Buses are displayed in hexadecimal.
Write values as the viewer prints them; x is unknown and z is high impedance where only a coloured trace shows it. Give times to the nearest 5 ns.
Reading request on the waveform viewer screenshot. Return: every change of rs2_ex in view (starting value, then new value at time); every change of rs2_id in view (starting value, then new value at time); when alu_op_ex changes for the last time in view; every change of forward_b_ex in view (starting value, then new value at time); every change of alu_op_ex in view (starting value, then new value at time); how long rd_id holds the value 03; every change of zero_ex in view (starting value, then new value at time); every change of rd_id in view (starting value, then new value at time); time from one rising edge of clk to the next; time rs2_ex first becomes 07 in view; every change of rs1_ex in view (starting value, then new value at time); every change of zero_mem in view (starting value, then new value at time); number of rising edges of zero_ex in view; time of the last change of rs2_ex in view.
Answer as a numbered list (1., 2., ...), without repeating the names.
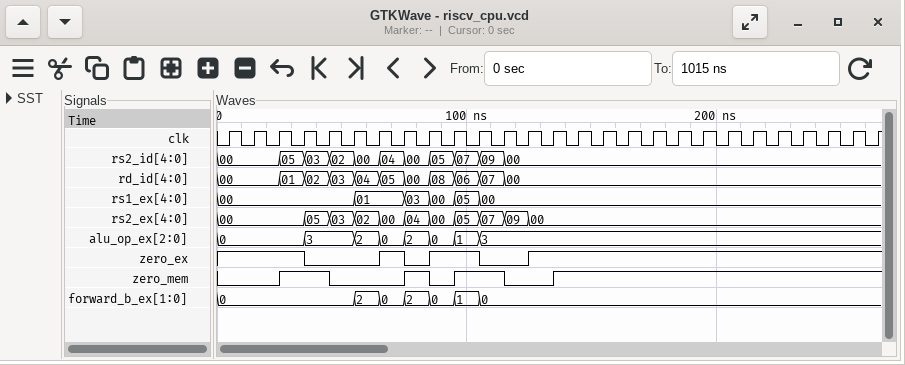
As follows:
1. 00, 05 at 35 ns, 03 at 45 ns, 02 at 55 ns, 00 at 65 ns, 04 at 75 ns, 00 at 85 ns, 05 at 95 ns, 07 at 105 ns, 09 at 115 ns, 00 at 125 ns
2. 00, 05 at 25 ns, 03 at 35 ns, 02 at 45 ns, 00 at 55 ns, 04 at 65 ns, 00 at 75 ns, 05 at 85 ns, 07 at 95 ns, 09 at 105 ns, 00 at 115 ns
3. 105 ns
4. 0, 2 at 55 ns, 0 at 65 ns, 2 at 75 ns, 0 at 85 ns, 1 at 95 ns, 0 at 105 ns
5. 0, 3 at 35 ns, 2 at 55 ns, 0 at 65 ns, 2 at 75 ns, 0 at 85 ns, 1 at 95 ns, 3 at 105 ns
6. 10 ns
7. 1, 0 at 35 ns, 1 at 65 ns, 0 at 75 ns, 1 at 85 ns, 0 at 105 ns, 1 at 125 ns
8. 00, 01 at 25 ns, 02 at 35 ns, 03 at 45 ns, 04 at 55 ns, 05 at 65 ns, 00 at 75 ns, 08 at 85 ns, 06 at 95 ns, 07 at 105 ns, 00 at 115 ns
9. 10 ns
10. 105 ns
11. 00, 01 at 55 ns, 03 at 75 ns, 00 at 85 ns, 05 at 95 ns, 00 at 105 ns
12. 0, 1 at 25 ns, 0 at 45 ns, 1 at 75 ns, 0 at 85 ns, 1 at 95 ns, 0 at 115 ns, 1 at 135 ns
13. 3
14. 125 ns
